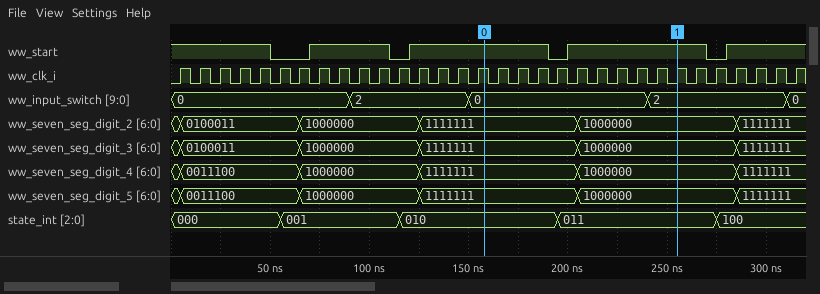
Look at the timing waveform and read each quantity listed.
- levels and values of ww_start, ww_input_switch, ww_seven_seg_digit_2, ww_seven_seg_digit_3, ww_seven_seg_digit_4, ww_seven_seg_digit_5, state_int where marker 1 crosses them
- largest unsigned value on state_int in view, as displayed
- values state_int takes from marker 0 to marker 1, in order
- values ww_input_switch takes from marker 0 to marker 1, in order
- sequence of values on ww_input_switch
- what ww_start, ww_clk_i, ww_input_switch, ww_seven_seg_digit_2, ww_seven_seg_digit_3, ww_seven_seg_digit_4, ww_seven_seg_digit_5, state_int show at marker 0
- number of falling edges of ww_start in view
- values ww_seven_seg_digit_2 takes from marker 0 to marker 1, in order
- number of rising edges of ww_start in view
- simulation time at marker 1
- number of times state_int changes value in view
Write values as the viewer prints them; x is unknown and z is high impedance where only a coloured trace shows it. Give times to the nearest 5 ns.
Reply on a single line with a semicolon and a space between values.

ww_start=1, ww_input_switch=2, ww_seven_seg_digit_2=1000000, ww_seven_seg_digit_3=1000000, ww_seven_seg_digit_4=1000000, ww_seven_seg_digit_5=1000000, state_int=011; 100; 010, 011; 0, 2; 0, 2, 0, 2, 0; ww_start=1, ww_clk_i=1, ww_input_switch=0, ww_seven_seg_digit_2=1111111, ww_seven_seg_digit_3=1111111, ww_seven_seg_digit_4=1111111, ww_seven_seg_digit_5=1111111, state_int=010; 4; 1111111, 1000000; 4; 255 ns; 4
